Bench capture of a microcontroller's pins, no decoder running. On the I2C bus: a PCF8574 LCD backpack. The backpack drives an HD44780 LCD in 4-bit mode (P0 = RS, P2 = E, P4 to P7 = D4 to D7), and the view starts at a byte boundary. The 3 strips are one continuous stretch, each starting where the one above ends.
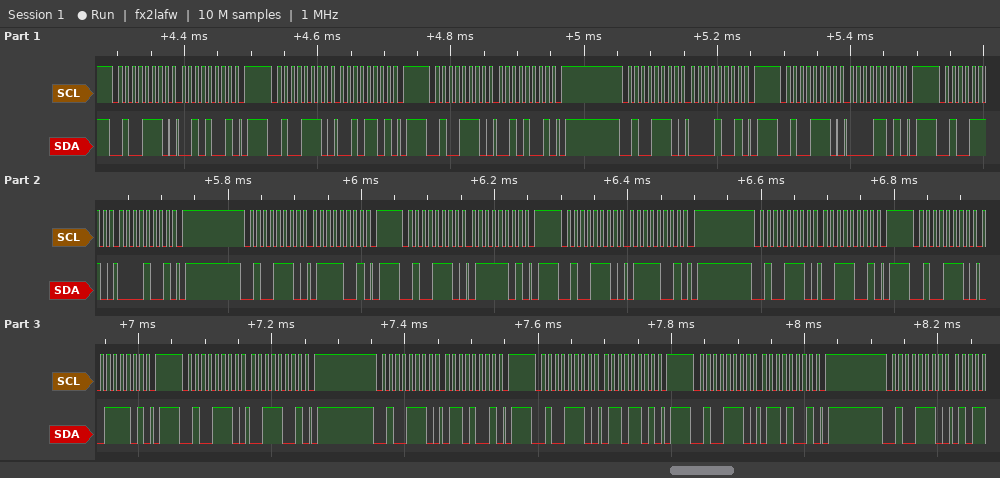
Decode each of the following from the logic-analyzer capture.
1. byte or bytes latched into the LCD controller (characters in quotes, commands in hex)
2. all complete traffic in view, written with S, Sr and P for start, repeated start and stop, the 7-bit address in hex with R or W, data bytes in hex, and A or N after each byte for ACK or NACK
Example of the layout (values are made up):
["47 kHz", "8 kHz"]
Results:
["' ' 's'", "S 27W A 29 A P S 27W A 2D A P S 27W A 29 A P S 27W A 09 A P S 27W A 0D A P S 27W A 09 A P S 27W A 79 A P S 27W A 7D A P S 27W A 79 A P S 27W A 39 A P S 27W A 3D A P S 27W A 39 A P S 27W A 69 A P S 27W A 6D A P S 27W A 69 A P S 27W A"]
